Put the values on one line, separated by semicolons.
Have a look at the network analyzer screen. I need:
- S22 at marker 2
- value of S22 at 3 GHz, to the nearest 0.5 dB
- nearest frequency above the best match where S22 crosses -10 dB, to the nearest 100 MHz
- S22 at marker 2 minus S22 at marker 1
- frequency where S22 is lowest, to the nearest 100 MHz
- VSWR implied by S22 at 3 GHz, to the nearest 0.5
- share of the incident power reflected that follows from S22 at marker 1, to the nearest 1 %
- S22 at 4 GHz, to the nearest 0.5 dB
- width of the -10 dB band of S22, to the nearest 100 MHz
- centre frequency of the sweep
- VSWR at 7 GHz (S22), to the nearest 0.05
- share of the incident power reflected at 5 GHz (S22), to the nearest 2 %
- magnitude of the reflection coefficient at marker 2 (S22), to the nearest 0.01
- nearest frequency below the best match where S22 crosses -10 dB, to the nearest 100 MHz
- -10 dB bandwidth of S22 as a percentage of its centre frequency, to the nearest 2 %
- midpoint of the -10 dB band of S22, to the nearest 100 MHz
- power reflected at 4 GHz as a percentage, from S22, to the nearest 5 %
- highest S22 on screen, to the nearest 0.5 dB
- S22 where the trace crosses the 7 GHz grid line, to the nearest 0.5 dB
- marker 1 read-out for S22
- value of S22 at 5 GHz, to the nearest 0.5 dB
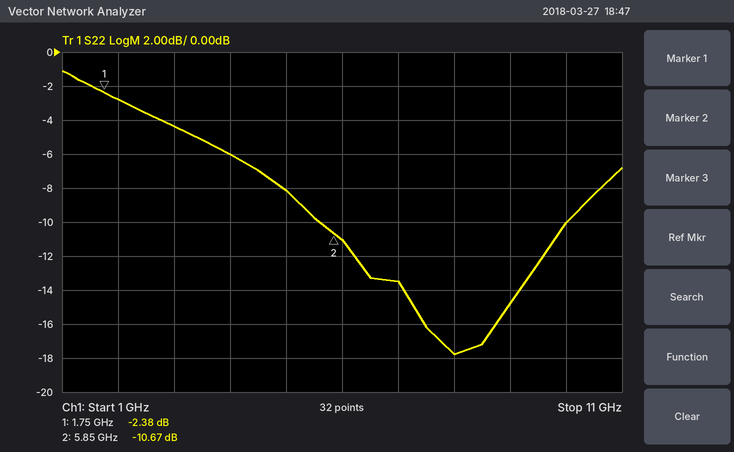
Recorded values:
-10.67 dB; -4.5 dB; 10.0 GHz; -8.29 dB; 8.0 GHz; 4.0; 58 %; -6.0 dB; 4.4 GHz; 6 GHz; 1.55; 16 %; 0.29; 5.6 GHz; 56 %; 7.8 GHz; 25 %; -1.0 dB; -13.5 dB; -2.38 dB; -8.0 dB
